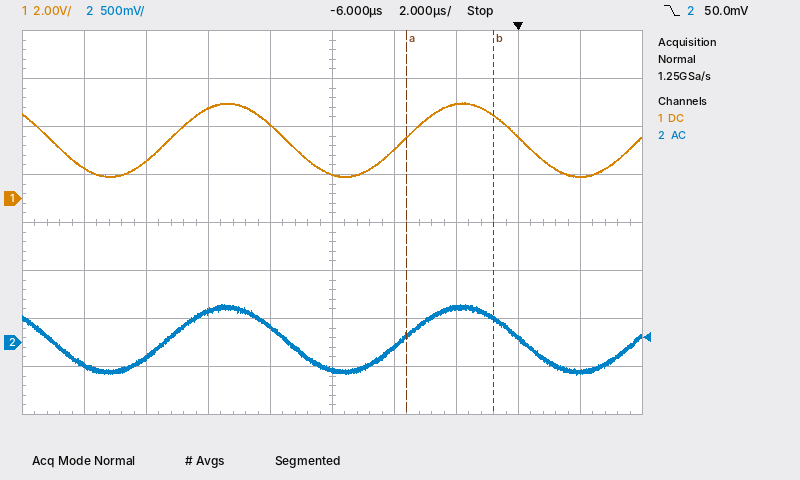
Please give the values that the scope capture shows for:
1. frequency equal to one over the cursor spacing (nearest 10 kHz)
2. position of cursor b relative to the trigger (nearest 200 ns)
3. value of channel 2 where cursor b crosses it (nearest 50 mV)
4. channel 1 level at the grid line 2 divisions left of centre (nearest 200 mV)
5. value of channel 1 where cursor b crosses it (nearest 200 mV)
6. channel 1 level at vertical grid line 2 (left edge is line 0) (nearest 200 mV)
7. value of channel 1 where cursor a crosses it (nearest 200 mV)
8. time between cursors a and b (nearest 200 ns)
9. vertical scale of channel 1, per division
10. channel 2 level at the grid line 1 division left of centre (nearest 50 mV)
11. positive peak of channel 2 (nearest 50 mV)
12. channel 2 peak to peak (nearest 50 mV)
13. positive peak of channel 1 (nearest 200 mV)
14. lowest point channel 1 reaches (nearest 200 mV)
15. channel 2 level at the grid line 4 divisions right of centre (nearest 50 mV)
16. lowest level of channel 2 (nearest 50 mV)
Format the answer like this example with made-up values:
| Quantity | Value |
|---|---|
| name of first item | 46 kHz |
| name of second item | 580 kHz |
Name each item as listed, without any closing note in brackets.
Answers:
| Quantity | Value |
|---|---|
| frequency equal to one over the cursor spacing | 360 kHz |
| position of cursor b relative to the trigger | -800 ns |
| value of channel 2 where cursor b crosses it | 250 mV |
| channel 1 level at the grid line 2 divisions left of centre | 3.8 V |
| value of channel 1 where cursor b crosses it | 3.4 V |
| channel 1 level at vertical grid line 2 (left edge is line 0) | 1.6 V |
| value of channel 1 where cursor a crosses it | 2.6 V |
| time between cursors a and b | 2.8 µs |
| vertical scale of channel 1, per division | 2 V |
| channel 2 level at the grid line 1 division left of centre | 150 mV |
| positive peak of channel 2 | 400 mV |
| channel 2 peak to peak | 750 mV |
| positive peak of channel 1 | 4.0 V |
| lowest point channel 1 reaches | 800 mV |
| channel 2 level at the grid line 4 divisions right of centre | -300 mV |
| lowest level of channel 2 | -350 mV |
